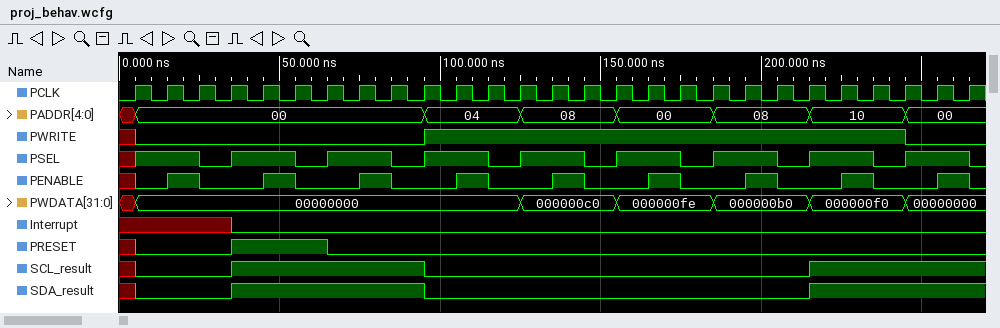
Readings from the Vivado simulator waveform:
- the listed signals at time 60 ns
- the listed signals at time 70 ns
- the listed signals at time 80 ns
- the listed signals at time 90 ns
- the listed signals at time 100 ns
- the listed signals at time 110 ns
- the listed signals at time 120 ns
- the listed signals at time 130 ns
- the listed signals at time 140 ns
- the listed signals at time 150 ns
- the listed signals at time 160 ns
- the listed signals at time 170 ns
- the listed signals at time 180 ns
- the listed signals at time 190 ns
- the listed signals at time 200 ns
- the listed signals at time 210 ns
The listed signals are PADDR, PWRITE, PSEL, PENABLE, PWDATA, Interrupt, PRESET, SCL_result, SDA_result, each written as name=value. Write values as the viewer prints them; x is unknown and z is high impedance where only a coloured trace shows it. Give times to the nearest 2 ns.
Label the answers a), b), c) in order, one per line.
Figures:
a) PADDR=00, PWRITE=0, PSEL=0, PENABLE=0, PWDATA=00000000, Interrupt=0, PRESET=1, SCL_result=1, SDA_result=1
b) PADDR=00, PWRITE=0, PSEL=1, PENABLE=0, PWDATA=00000000, Interrupt=0, PRESET=0, SCL_result=1, SDA_result=1
c) PADDR=00, PWRITE=0, PSEL=1, PENABLE=1, PWDATA=00000000, Interrupt=0, PRESET=0, SCL_result=1, SDA_result=1
d) PADDR=00, PWRITE=0, PSEL=0, PENABLE=0, PWDATA=00000000, Interrupt=0, PRESET=0, SCL_result=1, SDA_result=1
e) PADDR=04, PWRITE=1, PSEL=1, PENABLE=0, PWDATA=00000000, Interrupt=0, PRESET=0, SCL_result=0, SDA_result=0
f) PADDR=04, PWRITE=1, PSEL=1, PENABLE=1, PWDATA=00000000, Interrupt=0, PRESET=0, SCL_result=0, SDA_result=0
g) PADDR=04, PWRITE=1, PSEL=0, PENABLE=0, PWDATA=00000000, Interrupt=0, PRESET=0, SCL_result=0, SDA_result=0
h) PADDR=08, PWRITE=1, PSEL=1, PENABLE=0, PWDATA=000000c0, Interrupt=0, PRESET=0, SCL_result=0, SDA_result=0
i) PADDR=08, PWRITE=1, PSEL=1, PENABLE=1, PWDATA=000000c0, Interrupt=0, PRESET=0, SCL_result=0, SDA_result=0
j) PADDR=08, PWRITE=1, PSEL=0, PENABLE=0, PWDATA=000000c0, Interrupt=0, PRESET=0, SCL_result=0, SDA_result=0
k) PADDR=00, PWRITE=1, PSEL=1, PENABLE=0, PWDATA=000000fe, Interrupt=0, PRESET=0, SCL_result=0, SDA_result=0
l) PADDR=00, PWRITE=1, PSEL=1, PENABLE=1, PWDATA=000000fe, Interrupt=0, PRESET=0, SCL_result=0, SDA_result=0
m) PADDR=00, PWRITE=1, PSEL=0, PENABLE=0, PWDATA=000000fe, Interrupt=0, PRESET=0, SCL_result=0, SDA_result=0
n) PADDR=08, PWRITE=1, PSEL=1, PENABLE=0, PWDATA=000000b0, Interrupt=0, PRESET=0, SCL_result=0, SDA_result=0
o) PADDR=08, PWRITE=1, PSEL=1, PENABLE=1, PWDATA=000000b0, Interrupt=0, PRESET=0, SCL_result=0, SDA_result=0
p) PADDR=08, PWRITE=1, PSEL=0, PENABLE=0, PWDATA=000000b0, Interrupt=0, PRESET=0, SCL_result=0, SDA_result=0
